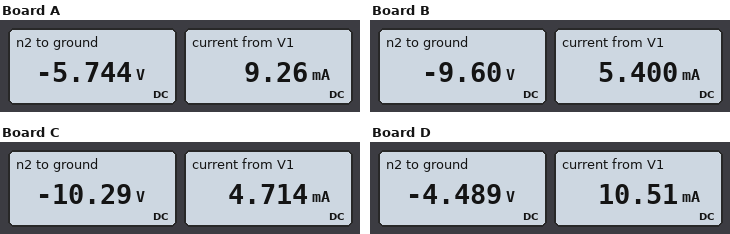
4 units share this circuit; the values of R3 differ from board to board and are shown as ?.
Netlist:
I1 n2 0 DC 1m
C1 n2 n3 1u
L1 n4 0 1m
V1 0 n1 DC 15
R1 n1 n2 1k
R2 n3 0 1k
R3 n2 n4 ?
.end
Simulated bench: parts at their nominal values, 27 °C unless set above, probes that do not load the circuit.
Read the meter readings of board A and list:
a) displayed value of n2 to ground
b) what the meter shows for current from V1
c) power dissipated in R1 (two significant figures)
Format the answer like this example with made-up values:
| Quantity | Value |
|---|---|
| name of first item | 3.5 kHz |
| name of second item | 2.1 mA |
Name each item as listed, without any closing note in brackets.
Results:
| Quantity | Value |
|---|---|
| displayed value of n2 to ground | -5.744 V |
| what the meter shows for current from V1 | 9.26 mA |
| power dissipated in R1 | 86 mW |
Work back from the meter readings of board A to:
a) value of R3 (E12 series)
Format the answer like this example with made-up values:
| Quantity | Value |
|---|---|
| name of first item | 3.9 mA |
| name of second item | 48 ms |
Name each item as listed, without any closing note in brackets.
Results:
| Quantity | Value |
|---|---|
| value of R3 | 560 Ω |
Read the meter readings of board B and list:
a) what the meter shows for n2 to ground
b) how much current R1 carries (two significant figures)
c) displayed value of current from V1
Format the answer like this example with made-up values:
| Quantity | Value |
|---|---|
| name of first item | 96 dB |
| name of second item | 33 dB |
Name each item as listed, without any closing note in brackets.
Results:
| Quantity | Value |
|---|---|
| what the meter shows for n2 to ground | -9.60 V |
| how much current R1 carries | 5.4 mA |
| displayed value of current from V1 | 5.400 mA |
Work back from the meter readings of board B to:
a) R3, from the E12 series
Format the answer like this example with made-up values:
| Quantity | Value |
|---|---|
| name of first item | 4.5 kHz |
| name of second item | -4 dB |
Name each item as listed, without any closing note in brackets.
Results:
| Quantity | Value |
|---|---|
| R3, from the E12 series | 1.5 kΩ |
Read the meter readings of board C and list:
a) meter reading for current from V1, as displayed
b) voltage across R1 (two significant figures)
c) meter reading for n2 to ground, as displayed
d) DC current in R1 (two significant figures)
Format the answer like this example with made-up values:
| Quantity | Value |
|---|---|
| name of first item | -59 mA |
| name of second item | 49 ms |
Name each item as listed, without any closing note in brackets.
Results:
| Quantity | Value |
|---|---|
| meter reading for current from V1, as displayed | 4.714 mA |
| voltage across R1 | 4.7 V |
| meter reading for n2 to ground, as displayed | -10.29 V |
| DC current in R1 | 4.7 mA |
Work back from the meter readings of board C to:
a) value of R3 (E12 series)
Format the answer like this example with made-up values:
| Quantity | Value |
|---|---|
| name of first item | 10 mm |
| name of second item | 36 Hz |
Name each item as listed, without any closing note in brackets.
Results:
| Quantity | Value |
|---|---|
| value of R3 | 1.8 kΩ |
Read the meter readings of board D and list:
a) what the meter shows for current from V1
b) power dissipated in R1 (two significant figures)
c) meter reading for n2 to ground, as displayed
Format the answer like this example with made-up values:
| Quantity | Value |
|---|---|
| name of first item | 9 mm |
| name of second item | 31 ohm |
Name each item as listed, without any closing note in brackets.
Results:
| Quantity | Value |
|---|---|
| what the meter shows for current from V1 | 10.51 mA |
| power dissipated in R1 | 110 mW |
| meter reading for n2 to ground, as displayed | -4.489 V |
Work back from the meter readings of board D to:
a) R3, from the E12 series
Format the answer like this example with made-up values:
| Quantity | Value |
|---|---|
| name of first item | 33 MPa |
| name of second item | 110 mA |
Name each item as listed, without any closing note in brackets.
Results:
| Quantity | Value |
|---|---|
| R3, from the E12 series | 390 Ω |
